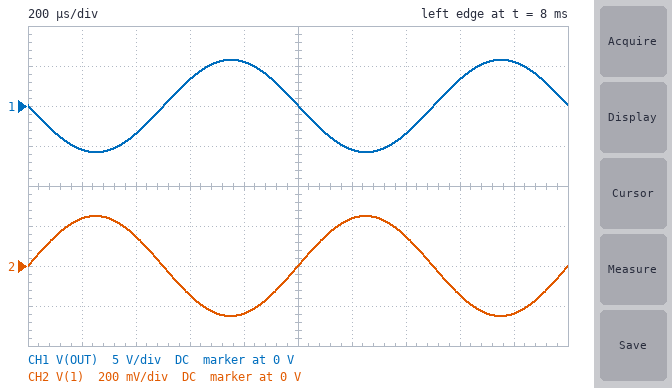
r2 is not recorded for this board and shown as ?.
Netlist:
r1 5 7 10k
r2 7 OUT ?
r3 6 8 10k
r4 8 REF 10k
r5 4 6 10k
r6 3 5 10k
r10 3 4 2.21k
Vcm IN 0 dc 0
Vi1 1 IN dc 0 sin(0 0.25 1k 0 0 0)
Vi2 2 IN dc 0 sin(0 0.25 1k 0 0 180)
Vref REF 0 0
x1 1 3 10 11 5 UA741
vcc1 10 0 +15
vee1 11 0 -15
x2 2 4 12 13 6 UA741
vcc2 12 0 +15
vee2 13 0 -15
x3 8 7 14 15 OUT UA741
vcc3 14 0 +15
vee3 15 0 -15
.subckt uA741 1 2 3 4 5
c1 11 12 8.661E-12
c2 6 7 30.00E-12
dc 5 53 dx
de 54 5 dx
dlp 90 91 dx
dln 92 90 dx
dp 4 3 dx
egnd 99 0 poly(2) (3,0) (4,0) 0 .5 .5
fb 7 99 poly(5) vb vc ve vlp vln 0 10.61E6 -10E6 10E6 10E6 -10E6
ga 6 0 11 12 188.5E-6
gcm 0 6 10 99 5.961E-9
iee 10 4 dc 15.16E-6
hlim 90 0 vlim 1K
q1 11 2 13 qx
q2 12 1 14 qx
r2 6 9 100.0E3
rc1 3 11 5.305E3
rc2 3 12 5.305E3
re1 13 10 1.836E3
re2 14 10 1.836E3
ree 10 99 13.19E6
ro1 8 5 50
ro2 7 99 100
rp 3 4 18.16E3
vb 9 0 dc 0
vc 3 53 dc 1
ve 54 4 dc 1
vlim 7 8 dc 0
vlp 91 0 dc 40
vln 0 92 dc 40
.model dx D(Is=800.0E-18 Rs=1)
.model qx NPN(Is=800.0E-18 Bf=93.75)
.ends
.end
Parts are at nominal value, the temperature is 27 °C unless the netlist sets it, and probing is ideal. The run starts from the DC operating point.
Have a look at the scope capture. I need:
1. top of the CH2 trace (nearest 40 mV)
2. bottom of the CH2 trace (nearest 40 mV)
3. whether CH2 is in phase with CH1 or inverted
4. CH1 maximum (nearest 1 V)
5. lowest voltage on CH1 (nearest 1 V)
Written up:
240 mV
-240 mV
inverted
6 V
-6 V
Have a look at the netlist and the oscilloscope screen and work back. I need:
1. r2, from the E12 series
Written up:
12 kΩ
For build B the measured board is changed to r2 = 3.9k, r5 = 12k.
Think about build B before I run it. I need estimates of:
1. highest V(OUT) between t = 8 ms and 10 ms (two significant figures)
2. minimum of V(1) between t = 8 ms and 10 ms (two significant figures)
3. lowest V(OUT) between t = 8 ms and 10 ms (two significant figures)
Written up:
3.0 V
-250 mV
-3.0 V
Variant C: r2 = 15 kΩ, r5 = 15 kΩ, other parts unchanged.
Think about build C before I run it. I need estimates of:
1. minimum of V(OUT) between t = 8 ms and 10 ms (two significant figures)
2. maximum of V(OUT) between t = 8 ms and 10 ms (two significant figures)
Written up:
-8.3 V
8.3 V
